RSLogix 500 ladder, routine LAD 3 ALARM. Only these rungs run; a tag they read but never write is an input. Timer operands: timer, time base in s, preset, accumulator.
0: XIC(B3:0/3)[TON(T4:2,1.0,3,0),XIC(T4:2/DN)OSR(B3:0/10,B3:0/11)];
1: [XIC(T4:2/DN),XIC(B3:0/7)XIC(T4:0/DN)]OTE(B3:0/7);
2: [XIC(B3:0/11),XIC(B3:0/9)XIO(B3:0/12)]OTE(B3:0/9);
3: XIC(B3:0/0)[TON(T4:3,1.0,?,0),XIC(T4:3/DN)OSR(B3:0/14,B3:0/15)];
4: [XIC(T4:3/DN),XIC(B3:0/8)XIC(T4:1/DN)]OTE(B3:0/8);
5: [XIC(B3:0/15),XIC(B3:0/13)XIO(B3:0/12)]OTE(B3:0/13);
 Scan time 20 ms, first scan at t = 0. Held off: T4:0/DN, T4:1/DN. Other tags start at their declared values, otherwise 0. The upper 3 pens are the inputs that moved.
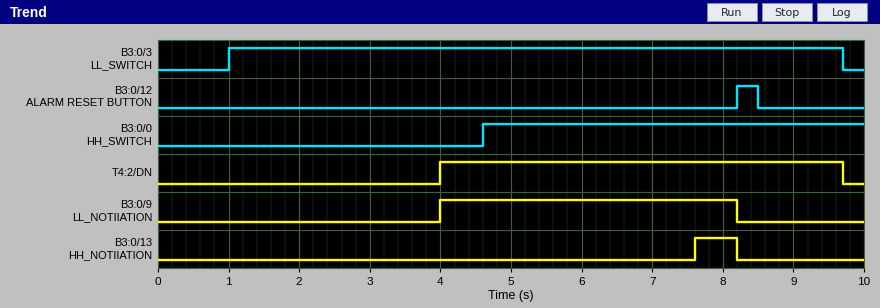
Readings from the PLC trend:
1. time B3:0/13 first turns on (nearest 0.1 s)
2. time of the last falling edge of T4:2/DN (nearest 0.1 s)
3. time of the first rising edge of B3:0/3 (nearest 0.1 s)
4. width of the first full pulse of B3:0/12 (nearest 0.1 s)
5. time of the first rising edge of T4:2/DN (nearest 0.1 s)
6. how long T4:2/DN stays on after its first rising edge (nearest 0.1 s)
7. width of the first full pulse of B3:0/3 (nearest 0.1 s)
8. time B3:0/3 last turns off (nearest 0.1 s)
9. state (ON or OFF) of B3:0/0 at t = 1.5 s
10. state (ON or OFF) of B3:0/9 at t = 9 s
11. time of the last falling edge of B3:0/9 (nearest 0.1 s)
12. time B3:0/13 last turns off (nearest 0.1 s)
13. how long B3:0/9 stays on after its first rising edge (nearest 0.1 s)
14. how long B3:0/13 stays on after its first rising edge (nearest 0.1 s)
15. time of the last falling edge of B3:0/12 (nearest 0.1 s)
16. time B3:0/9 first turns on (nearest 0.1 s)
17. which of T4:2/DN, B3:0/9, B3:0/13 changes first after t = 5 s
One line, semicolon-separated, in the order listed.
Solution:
7.6 s; 9.7 s; 1.0 s; 0.3 s; 4.0 s; 5.7 s; 8.7 s; 9.7 s; OFF; OFF; 8.2 s; 8.2 s; 4.2 s; 0.6 s; 8.5 s; 4.0 s; B3:0/13
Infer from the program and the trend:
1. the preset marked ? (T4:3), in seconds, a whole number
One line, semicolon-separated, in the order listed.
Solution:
3 s
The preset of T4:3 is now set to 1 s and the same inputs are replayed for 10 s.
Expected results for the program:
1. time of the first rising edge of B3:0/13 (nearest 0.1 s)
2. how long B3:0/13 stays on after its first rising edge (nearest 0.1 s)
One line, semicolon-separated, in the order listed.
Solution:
5.6 s; 2.6 s
